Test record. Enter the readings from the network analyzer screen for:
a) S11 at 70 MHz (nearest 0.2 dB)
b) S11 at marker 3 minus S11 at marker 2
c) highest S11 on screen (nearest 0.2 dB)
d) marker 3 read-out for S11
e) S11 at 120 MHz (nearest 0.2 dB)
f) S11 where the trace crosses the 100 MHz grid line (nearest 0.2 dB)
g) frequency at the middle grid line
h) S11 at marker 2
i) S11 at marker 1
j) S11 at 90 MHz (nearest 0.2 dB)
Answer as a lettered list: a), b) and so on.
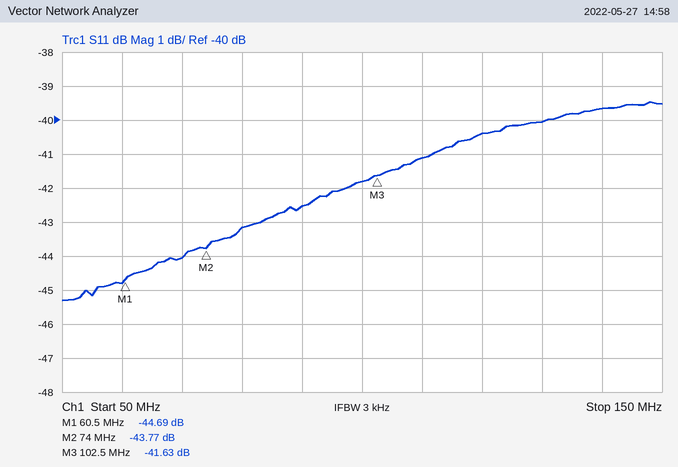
a) -44.0 dB
b) 2.14 dB
c) -39.4 dB
d) -41.63 dB
e) -40.4 dB
f) -41.8 dB
g) 100 MHz
h) -43.77 dB
i) -44.69 dB
j) -42.6 dB
